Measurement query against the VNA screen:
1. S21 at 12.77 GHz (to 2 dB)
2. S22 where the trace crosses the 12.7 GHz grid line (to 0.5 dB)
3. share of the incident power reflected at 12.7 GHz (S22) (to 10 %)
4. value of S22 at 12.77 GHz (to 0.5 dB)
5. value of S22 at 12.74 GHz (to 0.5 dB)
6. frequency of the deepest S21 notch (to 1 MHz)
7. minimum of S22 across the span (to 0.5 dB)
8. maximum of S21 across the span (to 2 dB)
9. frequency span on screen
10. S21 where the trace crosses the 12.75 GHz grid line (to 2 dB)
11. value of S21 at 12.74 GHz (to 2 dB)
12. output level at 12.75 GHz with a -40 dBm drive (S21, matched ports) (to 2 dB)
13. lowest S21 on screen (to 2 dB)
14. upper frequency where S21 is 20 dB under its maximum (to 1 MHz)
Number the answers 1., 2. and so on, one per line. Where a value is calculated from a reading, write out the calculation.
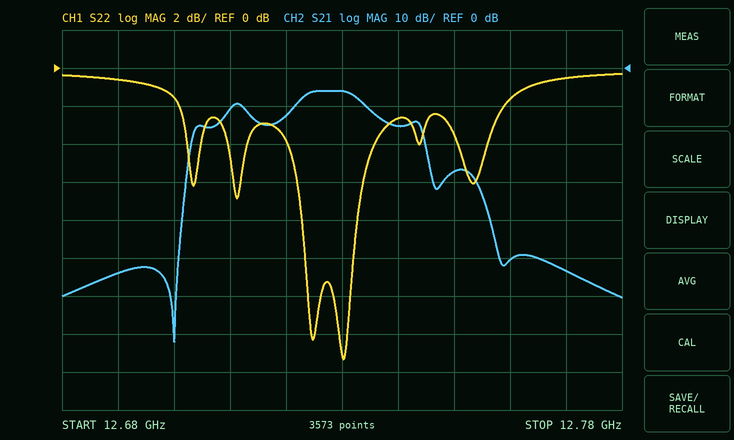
1. -54 dB
2. -1.5 dB
3. 10^(-1.5/10) ≈ 70.8 %, so 70 % to the nearest 10 %
4. -0.5 dB
5. -2.5 dB
6. 12.700 GHz
7. -15.5 dB
8. -6 dB
9. 100 MHz
10. -28 dB
11. -16 dB
12. -40 dBm + (-28 dB) = -68 dBm
13. -72 dB
14. 12.746 GHz
